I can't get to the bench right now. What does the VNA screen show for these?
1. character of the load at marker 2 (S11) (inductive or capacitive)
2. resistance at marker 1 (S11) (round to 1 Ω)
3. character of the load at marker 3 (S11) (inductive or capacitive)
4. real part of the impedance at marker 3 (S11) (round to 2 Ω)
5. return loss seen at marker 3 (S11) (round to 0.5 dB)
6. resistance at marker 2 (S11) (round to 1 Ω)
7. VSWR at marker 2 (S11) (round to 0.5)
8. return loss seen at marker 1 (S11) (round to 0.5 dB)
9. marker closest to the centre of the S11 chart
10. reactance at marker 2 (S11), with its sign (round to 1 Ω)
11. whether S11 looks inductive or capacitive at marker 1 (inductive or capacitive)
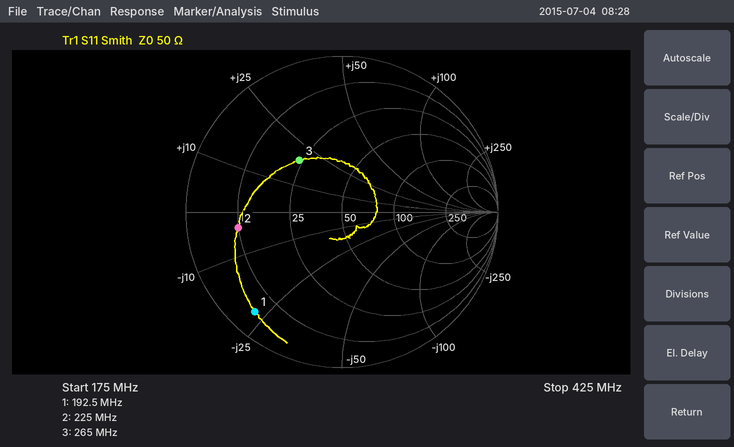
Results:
capacitive
5 Ω
inductive
24 Ω
7.5 dB
10 Ω
5.0
1.5 dB
marker 3
-4 Ω
capacitive
